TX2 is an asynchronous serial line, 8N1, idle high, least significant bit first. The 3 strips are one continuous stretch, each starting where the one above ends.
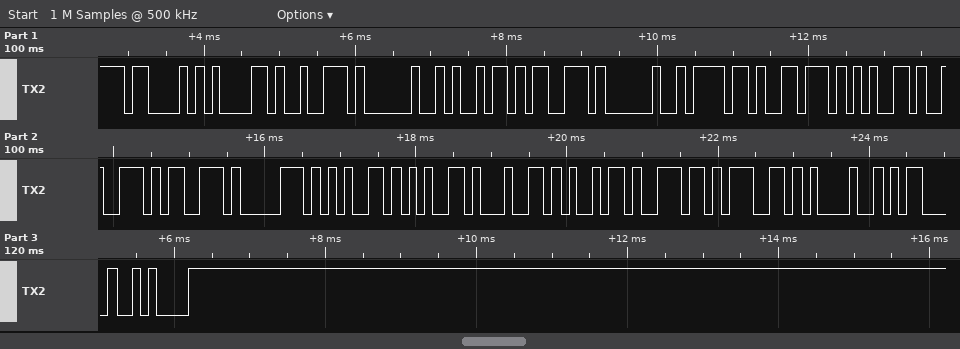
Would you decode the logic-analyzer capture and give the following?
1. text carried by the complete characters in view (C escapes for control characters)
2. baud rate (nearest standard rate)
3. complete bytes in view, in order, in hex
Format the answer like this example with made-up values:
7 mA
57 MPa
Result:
"Car is overspeeding!\r\n"
9600 baud
43 61 72 20 69 73 20 6F 76 65 72 73 70 65 65 64 69 6E 67 21 0D 0A
